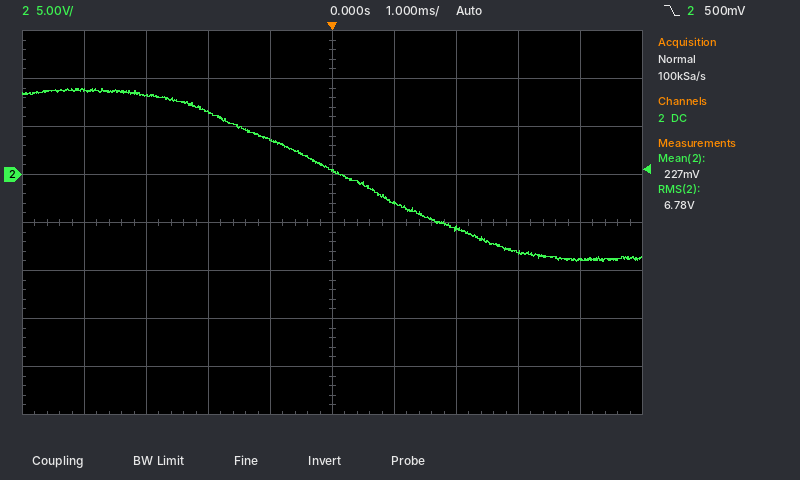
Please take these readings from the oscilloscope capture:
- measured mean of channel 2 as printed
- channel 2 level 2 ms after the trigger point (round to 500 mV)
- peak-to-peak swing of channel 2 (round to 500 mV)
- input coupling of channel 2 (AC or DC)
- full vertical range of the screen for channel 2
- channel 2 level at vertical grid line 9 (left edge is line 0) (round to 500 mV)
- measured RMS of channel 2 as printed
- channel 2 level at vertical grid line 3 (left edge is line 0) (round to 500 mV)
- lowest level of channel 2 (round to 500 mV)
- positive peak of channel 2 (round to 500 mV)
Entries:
227 mV
-5.5 V
18.0 V
DC
40 V
-9.0 V
6.78 V
6.5 V
-9.0 V
9.0 V
